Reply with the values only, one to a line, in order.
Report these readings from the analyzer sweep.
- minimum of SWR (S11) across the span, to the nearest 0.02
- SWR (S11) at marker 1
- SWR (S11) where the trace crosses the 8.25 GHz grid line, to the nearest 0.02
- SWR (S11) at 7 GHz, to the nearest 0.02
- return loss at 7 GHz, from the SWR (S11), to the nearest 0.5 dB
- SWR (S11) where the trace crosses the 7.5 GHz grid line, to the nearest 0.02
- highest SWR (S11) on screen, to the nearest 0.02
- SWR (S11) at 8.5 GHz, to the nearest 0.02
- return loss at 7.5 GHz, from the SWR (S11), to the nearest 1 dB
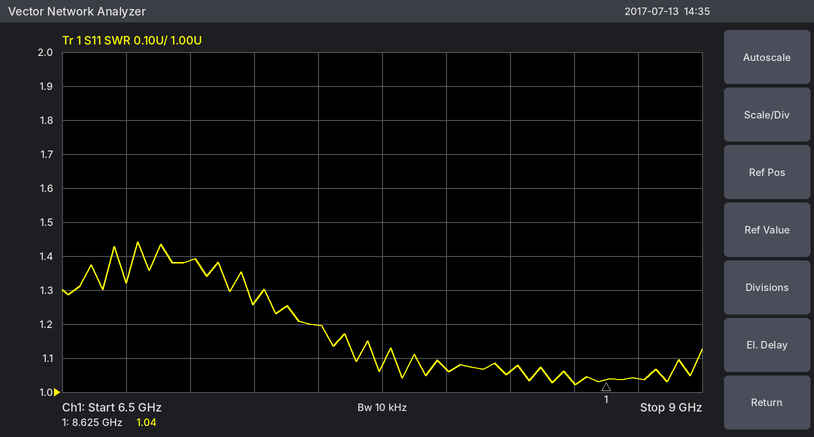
1.02
1.04
1.06
1.38
16.0 dB
1.20
1.44
1.02
21 dB
